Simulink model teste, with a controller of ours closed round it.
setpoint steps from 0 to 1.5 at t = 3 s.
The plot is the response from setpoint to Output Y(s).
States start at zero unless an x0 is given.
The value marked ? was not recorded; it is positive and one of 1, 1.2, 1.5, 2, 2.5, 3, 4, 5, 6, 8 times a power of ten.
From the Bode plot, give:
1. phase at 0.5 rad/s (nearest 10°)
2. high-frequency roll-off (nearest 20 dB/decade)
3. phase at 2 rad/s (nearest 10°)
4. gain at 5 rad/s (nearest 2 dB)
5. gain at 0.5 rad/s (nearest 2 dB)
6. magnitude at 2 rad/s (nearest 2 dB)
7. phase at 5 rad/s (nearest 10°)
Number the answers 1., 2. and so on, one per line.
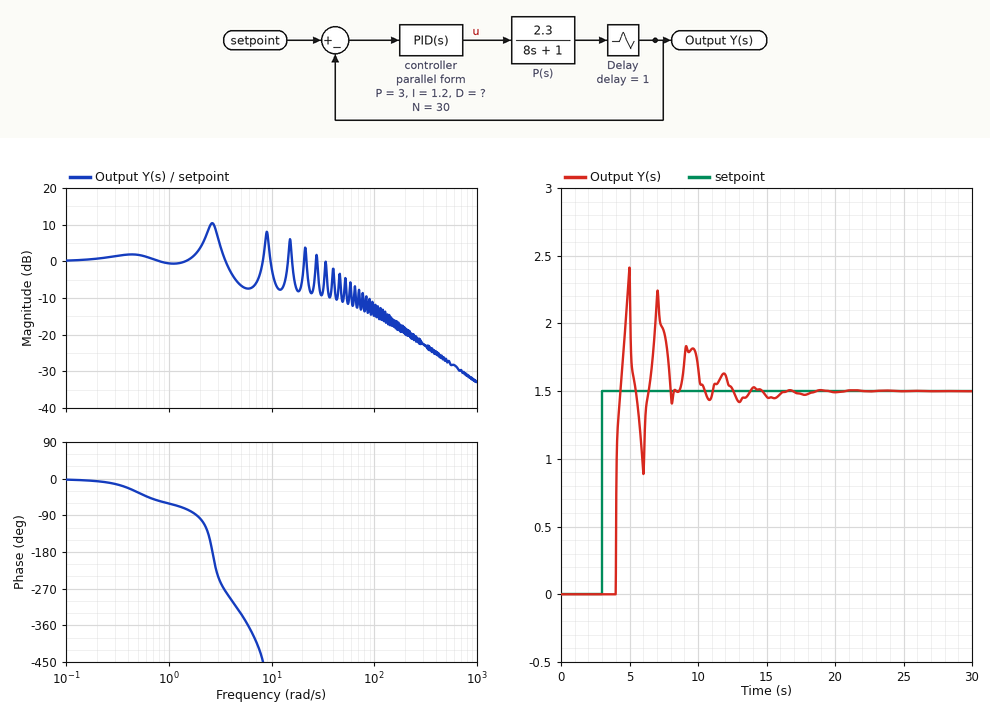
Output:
1. -30°
2. -20 dB/decade
3. -100°
4. -6 dB
5. 2 dB
6. 4 dB
7. -330°
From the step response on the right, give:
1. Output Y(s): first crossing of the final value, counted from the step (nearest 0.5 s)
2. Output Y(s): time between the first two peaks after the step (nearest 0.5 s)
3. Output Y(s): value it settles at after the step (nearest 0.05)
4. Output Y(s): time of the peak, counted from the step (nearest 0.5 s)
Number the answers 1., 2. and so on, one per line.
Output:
1. 1.5 s
2. 2.0 s
3. 1.50
4. 2.0 s
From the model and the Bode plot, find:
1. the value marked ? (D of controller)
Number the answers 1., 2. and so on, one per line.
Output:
1. 2.5
